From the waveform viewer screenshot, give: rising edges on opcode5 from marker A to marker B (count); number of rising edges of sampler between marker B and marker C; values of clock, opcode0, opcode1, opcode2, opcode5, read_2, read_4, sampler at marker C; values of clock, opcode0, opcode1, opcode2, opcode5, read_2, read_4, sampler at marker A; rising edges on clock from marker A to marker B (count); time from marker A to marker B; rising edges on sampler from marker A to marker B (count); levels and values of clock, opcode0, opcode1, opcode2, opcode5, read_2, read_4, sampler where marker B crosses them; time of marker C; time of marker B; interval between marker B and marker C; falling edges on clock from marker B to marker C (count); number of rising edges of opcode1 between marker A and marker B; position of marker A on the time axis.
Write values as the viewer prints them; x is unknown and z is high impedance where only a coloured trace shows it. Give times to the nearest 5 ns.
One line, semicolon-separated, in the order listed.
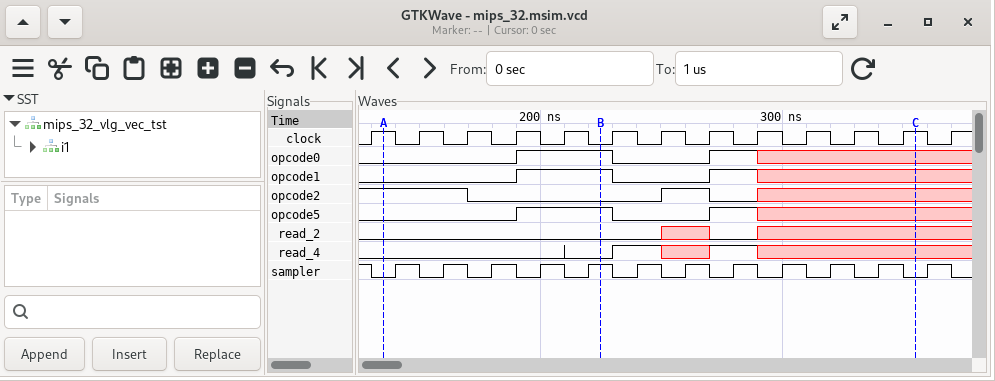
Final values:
1; 6; clock=1, opcode0=x, opcode1=x, opcode2=x, opcode5=x, read_2=x, read_4=x, sampler=0; clock=1, opcode0=0, opcode1=0, opcode2=1, opcode5=0, read_2=0, read_4=0, sampler=0; 4; 90 ns; 5; clock=0, opcode0=1, opcode1=1, opcode2=0, opcode5=1, read_2=0, read_4=0, sampler=1; 355 ns; 225 ns; 130 ns; 6; 1; 135 ns
